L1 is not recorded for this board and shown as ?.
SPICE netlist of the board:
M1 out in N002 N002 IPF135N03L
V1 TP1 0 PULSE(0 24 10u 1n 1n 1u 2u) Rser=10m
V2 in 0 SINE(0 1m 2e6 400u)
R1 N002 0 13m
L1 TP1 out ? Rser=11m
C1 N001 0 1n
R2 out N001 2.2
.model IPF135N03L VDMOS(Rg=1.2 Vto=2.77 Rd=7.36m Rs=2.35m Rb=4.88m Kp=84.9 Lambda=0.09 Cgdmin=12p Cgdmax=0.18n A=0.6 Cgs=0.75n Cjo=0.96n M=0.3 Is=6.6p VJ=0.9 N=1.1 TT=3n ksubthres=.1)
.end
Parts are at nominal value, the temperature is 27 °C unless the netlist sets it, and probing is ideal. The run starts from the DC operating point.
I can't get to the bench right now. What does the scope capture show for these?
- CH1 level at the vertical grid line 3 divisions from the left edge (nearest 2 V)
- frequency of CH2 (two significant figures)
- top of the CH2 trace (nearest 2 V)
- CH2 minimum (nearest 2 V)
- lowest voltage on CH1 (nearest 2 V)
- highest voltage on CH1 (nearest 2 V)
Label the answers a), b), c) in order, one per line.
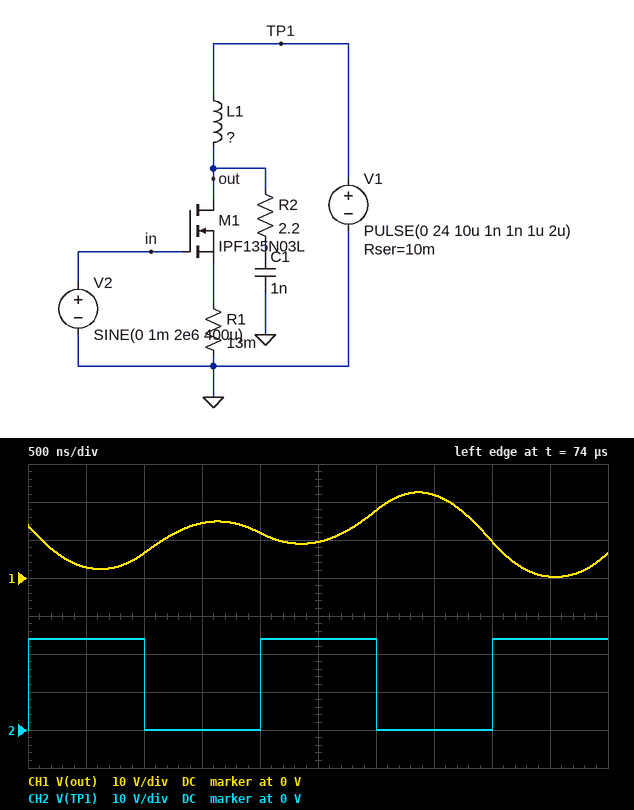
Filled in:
a) 14 V
b) 500 kHz
c) 24 V
d) 0 V
e) 0 V
f) 22 V
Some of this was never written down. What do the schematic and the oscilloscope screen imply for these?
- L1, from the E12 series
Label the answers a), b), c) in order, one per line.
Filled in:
a) 220 µH
